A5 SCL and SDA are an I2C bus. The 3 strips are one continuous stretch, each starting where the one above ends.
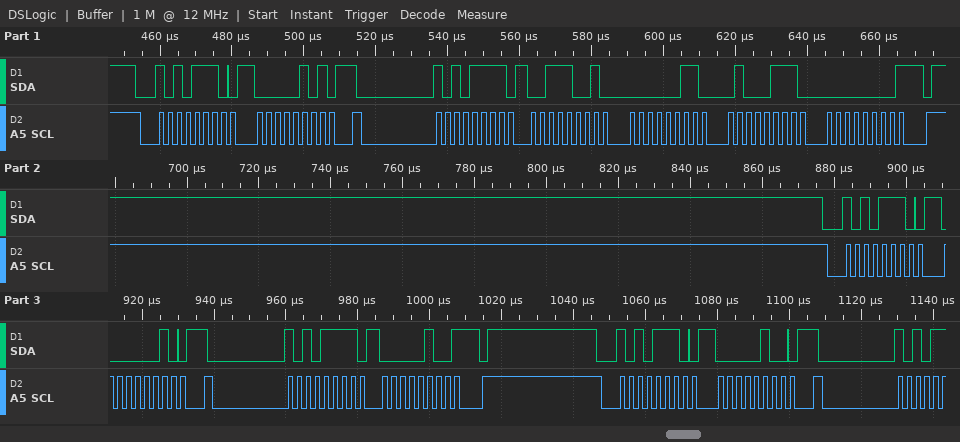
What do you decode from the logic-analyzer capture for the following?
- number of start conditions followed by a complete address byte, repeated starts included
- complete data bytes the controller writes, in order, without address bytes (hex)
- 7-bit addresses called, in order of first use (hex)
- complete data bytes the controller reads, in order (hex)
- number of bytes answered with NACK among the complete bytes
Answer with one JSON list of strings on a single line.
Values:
["5", "05 02 04", "0x57", "39 03 47 00 04", "2"]
